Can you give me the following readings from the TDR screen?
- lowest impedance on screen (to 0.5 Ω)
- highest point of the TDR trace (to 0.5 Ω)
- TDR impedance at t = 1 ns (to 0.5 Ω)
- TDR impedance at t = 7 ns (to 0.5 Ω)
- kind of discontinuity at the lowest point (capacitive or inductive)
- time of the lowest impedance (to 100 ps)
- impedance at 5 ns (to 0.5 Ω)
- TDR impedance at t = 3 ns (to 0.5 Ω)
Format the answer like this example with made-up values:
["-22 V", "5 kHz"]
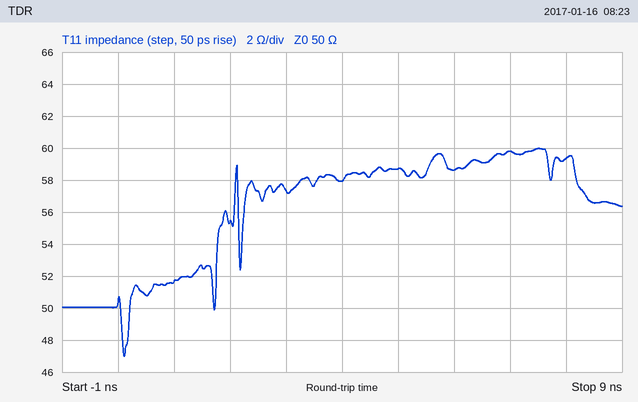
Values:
["47.0 Ω", "60.0 Ω", "51.5 Ω", "60.0 Ω", "capacitive", "100 ps", "58.5 Ω", "57.5 Ω"]
